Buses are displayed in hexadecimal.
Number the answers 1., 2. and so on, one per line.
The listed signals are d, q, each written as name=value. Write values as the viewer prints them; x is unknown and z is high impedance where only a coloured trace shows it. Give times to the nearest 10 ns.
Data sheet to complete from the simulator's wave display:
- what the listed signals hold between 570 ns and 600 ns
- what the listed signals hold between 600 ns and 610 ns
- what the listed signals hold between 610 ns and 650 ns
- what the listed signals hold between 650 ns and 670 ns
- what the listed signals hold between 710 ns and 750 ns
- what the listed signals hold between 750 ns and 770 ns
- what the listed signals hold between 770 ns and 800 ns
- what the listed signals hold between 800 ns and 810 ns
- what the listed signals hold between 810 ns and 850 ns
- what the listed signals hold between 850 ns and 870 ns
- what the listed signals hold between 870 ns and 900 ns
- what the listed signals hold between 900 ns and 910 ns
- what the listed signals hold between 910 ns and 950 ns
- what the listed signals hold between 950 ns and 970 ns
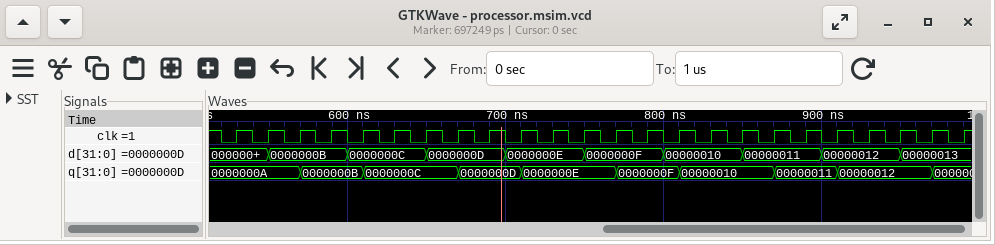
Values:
1. d=0000000B, q=0000000B
2. d=0000000C, q=0000000B
3. d=0000000C, q=0000000C
4. d=0000000D, q=0000000C
5. d=0000000E, q=0000000E
6. d=0000000F, q=0000000E
7. d=0000000F, q=0000000F
8. d=00000010, q=0000000F
9. d=00000010, q=00000010
10. d=00000011, q=00000010
11. d=00000011, q=00000011
12. d=00000012, q=00000011
13. d=00000012, q=00000012
14. d=00000013, q=00000012
